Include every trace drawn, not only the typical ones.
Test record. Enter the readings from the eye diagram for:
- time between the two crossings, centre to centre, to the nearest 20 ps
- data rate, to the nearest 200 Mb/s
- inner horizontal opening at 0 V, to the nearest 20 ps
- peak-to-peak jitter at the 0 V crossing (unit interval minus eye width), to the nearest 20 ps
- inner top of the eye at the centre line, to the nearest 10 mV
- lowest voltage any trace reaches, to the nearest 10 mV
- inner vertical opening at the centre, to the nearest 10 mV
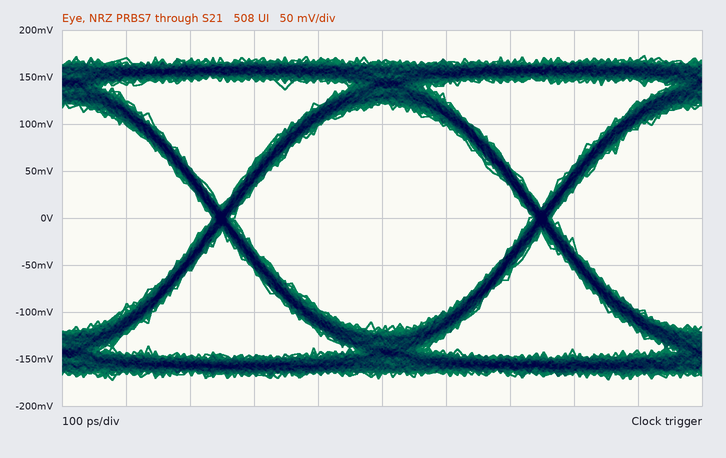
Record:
500 ps
2.0 Gb/s
460 ps
40 ps
120 mV
-170 mV
240 mV
